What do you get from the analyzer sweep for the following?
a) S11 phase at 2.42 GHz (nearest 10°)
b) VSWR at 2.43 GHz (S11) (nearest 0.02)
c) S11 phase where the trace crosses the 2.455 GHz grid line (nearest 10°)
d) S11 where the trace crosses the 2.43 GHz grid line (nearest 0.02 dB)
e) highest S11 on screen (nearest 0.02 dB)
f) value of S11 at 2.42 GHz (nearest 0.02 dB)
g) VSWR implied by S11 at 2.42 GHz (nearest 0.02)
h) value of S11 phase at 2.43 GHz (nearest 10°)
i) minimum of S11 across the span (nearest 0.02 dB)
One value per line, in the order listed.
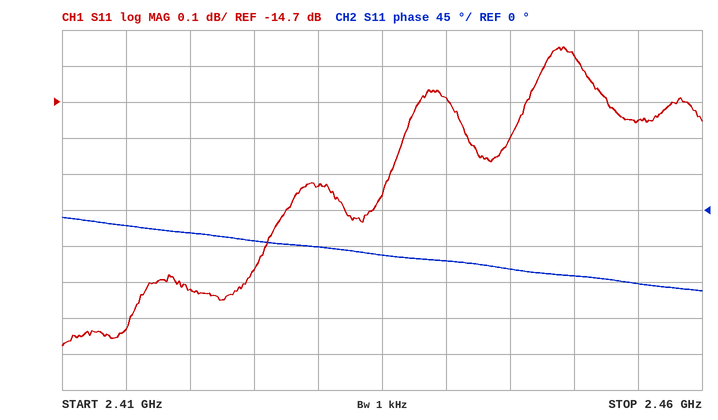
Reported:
-30°
1.44
-90°
-14.94 dB
-14.54 dB
-15.22 dB
1.42
-50°
-15.38 dB
